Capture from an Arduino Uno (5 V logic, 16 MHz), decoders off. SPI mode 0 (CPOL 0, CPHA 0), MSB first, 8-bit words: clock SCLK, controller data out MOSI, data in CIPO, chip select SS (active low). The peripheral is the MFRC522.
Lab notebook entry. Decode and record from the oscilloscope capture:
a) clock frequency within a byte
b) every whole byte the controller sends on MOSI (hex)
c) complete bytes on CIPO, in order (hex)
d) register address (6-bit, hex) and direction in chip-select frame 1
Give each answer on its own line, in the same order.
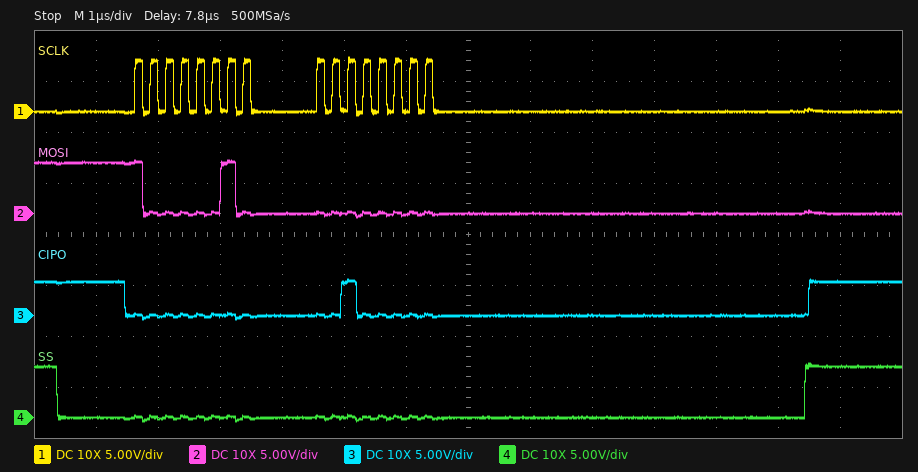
4 MHz
82 00
00 20
0x01 read
